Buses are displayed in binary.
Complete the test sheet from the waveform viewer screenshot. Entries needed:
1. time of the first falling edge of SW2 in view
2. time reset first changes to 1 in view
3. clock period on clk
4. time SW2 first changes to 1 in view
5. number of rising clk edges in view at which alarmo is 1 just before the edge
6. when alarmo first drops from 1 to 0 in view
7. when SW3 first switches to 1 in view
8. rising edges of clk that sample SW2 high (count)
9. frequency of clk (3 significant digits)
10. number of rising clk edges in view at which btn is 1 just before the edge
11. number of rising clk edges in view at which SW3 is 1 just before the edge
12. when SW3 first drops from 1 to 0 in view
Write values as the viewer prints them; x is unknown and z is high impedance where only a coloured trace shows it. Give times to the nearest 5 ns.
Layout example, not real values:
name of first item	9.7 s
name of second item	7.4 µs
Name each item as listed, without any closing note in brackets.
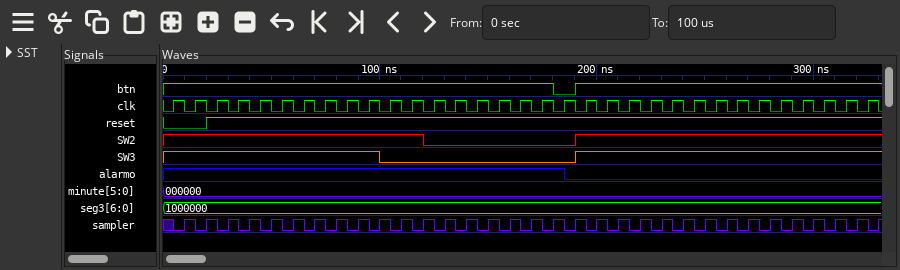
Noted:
time of the first falling edge of SW2 in view	120 ns
time reset first changes to 1 in view	20 ns
clock period on clk	10 ns
time SW2 first changes to 1 in view	190 ns
number of rising clk edges in view at which alarmo is 1 just before the edge	19
when alarmo first drops from 1 to 0 in view	185 ns
when SW3 first switches to 1 in view	190 ns
rising edges of clk that sample SW2 high	26
frequency of clk	100 MHz
number of rising clk edges in view at which btn is 1 just before the edge	32
number of rising clk edges in view at which SW3 is 1 just before the edge	24
when SW3 first drops from 1 to 0 in view	100 ns
